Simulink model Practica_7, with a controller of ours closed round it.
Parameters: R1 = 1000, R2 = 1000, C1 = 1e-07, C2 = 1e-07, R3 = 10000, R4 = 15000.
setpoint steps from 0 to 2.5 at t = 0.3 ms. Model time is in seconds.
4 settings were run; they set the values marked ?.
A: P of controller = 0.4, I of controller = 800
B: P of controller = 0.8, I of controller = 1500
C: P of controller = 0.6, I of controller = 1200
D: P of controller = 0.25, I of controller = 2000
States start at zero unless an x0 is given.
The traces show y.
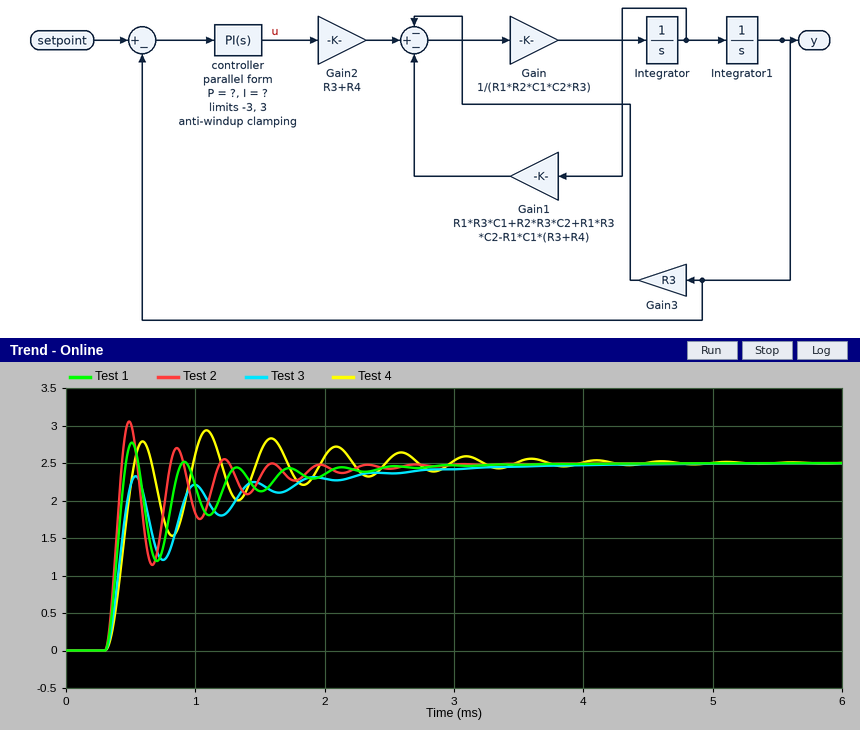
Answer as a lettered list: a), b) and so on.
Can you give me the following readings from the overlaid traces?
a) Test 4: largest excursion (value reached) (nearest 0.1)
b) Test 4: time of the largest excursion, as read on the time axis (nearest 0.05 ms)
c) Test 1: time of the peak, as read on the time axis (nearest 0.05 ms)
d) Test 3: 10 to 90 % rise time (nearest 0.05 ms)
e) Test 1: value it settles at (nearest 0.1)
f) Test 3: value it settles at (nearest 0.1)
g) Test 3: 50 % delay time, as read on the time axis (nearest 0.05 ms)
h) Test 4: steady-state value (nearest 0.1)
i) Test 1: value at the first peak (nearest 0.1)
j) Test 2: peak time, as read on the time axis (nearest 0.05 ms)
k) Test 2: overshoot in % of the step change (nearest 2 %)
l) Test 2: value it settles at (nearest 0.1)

a) 2.9
b) 1.10 ms
c) 0.50 ms
d) 0.15 ms
e) 2.5
f) 2.5
g) 0.40 ms
h) 2.5
i) 2.8
j) 0.50 ms
k) 22 %
l) 2.5
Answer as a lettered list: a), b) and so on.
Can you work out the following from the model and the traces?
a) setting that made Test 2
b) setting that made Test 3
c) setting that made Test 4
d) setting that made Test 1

a) B
b) A
c) D
d) C
